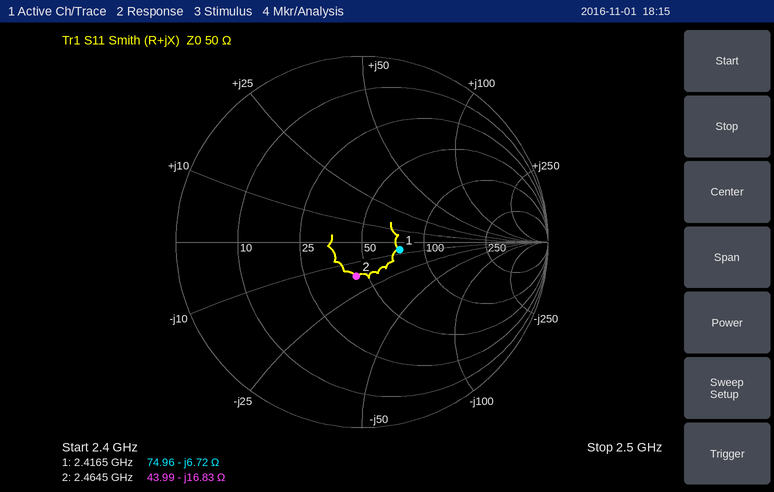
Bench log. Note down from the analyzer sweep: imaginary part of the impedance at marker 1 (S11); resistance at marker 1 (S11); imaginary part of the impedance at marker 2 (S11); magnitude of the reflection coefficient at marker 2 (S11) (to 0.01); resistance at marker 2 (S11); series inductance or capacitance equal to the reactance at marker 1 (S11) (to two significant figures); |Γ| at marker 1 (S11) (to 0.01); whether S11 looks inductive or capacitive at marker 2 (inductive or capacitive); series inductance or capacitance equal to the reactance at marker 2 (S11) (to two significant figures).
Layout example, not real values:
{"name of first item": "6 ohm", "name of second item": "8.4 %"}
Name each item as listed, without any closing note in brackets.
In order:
{"imaginary part of the impedance at marker 1": "-6.72 Ω", "resistance at marker 1": "74.96 Ω", "imaginary part of the impedance at marker 2": "-16.83 Ω", "magnitude of the reflection coefficient at marker 2 (S11)": "0.19", "resistance at marker 2": "43.99 Ω", "series inductance or capacitance equal to the reactance at marker 1 (S11)": "9.8 pF", "|Γ| at marker 1 (S11)": "0.21", "whether S11 looks inductive or capacitive at marker 2": "capacitive", "series inductance or capacitance equal to the reactance at marker 2 (S11)": "3.8 pF"}
